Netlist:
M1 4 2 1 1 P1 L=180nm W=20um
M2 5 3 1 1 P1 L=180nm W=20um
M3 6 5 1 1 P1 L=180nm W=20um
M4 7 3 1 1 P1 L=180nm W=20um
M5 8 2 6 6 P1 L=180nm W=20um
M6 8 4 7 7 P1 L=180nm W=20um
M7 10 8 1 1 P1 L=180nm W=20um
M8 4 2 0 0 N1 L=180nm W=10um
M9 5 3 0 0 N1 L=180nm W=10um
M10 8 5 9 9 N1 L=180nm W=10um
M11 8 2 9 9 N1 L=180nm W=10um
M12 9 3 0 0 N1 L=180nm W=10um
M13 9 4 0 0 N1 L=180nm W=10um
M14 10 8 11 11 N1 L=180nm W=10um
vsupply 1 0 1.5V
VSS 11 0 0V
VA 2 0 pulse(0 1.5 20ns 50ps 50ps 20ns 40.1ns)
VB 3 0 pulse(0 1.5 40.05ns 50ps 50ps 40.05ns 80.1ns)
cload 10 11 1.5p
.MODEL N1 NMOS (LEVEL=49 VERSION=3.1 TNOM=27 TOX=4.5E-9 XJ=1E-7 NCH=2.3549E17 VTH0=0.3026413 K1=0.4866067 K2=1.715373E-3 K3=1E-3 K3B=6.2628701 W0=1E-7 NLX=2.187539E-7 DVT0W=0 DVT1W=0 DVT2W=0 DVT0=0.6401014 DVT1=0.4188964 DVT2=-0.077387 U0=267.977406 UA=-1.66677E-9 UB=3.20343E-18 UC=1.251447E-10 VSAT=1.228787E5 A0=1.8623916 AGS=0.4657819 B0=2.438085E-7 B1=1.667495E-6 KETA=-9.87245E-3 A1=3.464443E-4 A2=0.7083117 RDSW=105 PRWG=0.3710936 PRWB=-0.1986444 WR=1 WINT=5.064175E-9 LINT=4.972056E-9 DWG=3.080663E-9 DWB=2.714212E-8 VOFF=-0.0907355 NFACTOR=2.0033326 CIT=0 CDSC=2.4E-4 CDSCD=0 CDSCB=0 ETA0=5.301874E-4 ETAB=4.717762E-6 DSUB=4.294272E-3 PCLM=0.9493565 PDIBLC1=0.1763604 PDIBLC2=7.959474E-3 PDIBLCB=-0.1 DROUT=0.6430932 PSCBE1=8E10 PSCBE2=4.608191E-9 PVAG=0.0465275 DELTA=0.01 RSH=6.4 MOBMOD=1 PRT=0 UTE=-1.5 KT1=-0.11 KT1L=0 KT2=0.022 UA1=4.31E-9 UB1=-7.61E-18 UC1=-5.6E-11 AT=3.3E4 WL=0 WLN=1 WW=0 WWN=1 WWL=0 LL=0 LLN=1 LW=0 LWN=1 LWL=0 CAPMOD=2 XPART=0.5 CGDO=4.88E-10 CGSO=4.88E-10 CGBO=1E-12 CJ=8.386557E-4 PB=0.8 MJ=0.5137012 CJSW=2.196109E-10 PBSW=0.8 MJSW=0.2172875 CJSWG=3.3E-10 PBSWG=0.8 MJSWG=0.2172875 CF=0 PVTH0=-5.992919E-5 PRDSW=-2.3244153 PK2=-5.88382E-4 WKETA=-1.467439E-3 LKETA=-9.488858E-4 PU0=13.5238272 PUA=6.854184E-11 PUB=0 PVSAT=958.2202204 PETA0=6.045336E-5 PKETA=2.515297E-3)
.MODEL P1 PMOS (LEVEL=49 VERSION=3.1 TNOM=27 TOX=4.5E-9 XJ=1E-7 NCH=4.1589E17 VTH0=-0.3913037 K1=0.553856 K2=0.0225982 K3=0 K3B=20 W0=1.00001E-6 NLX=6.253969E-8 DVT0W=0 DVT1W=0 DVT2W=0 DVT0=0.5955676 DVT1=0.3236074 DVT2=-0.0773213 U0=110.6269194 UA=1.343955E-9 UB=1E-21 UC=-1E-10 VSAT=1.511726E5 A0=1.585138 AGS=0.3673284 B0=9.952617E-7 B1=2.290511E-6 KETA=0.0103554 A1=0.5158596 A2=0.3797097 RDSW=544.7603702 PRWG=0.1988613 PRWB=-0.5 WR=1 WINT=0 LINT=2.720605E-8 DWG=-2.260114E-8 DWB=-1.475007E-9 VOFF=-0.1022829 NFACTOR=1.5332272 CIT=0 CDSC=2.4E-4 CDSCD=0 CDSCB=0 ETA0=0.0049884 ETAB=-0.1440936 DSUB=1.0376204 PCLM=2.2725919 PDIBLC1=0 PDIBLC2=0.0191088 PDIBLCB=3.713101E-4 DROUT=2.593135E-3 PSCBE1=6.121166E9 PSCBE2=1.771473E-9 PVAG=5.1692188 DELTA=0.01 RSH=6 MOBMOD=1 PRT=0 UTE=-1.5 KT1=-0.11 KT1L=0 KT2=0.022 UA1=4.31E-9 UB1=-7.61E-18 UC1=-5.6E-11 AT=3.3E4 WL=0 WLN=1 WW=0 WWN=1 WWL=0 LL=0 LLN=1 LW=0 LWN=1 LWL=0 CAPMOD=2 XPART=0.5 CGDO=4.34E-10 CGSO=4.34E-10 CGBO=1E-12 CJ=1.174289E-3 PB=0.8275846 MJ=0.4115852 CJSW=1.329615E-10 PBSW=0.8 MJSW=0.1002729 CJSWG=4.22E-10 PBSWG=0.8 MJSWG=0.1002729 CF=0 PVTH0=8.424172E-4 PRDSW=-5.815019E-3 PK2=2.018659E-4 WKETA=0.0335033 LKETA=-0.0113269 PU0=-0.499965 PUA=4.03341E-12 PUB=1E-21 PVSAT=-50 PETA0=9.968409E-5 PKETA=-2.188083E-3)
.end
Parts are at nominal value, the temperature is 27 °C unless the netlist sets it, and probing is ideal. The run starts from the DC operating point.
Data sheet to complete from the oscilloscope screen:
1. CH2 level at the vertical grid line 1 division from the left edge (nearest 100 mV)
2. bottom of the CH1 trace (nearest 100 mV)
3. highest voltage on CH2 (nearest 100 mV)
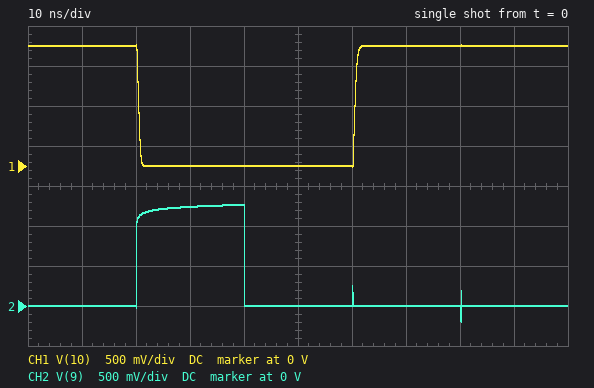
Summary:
0 V
0 V
1.3 V
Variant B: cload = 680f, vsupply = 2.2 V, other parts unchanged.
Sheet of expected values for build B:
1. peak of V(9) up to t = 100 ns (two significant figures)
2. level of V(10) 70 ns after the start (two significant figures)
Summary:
1.9 V
2.2 V
